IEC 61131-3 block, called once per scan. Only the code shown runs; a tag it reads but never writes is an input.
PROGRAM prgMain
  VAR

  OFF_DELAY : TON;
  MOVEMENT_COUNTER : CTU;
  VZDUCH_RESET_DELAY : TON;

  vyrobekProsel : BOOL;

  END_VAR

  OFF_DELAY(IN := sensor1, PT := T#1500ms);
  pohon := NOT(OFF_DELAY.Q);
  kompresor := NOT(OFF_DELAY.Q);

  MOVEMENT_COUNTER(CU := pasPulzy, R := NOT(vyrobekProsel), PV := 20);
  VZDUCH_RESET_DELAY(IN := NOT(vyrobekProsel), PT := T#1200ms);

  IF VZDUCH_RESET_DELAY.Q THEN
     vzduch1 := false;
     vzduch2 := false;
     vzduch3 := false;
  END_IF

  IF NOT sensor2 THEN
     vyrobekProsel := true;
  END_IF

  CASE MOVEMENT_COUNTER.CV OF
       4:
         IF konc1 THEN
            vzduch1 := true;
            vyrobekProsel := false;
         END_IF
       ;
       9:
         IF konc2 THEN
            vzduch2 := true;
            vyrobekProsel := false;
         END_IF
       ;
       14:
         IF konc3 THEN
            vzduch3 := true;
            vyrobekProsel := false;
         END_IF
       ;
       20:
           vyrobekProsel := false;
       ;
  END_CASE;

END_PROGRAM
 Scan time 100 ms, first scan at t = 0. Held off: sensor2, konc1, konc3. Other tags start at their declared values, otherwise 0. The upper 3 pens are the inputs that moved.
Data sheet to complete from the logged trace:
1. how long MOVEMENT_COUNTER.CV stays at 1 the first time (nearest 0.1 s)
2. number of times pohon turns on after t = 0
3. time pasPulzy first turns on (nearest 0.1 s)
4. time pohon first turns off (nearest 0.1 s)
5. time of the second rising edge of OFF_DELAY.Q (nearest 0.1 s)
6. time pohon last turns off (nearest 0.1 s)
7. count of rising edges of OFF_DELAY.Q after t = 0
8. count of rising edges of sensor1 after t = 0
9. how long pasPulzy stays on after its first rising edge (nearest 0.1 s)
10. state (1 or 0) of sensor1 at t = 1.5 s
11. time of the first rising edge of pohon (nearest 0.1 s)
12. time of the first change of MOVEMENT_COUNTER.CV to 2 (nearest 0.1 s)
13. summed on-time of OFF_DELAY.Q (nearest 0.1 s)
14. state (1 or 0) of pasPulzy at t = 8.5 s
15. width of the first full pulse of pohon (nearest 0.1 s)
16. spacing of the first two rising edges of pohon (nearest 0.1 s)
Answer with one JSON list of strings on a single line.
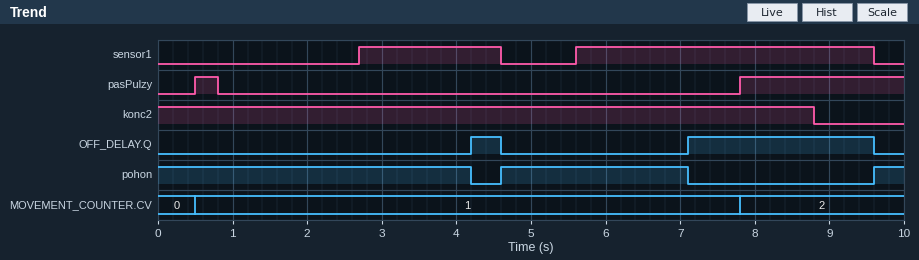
["7.3 s", "2", "0.5 s", "4.2 s", "7.1 s", "7.1 s", "2", "2", "0.3 s", "0", "4.6 s", "7.8 s", "2.9 s", "1", "2.5 s", "5.0 s"]
